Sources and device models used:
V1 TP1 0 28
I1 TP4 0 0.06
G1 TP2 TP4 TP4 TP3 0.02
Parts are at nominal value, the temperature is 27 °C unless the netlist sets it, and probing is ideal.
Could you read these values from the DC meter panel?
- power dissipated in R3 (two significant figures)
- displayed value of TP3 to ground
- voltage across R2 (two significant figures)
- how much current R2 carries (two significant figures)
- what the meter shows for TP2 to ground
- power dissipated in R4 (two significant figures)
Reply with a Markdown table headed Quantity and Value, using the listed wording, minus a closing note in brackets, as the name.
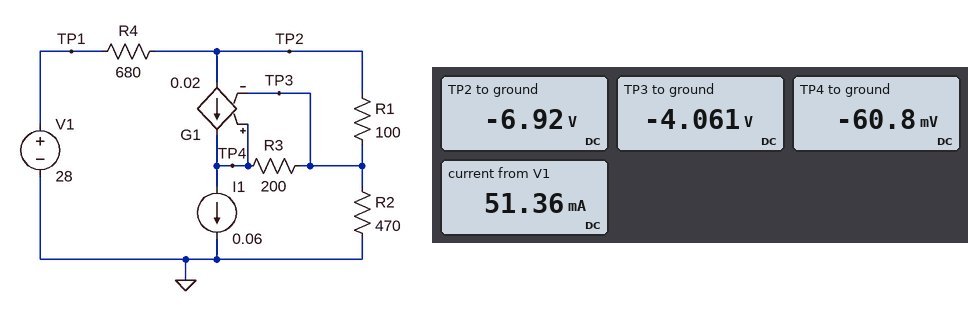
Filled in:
| Quantity | Value |
|---|---|
| power dissipated in R3 | 80 mW |
| displayed value of TP3 to ground | -4.061 V |
| voltage across R2 | 4.1 V |
| how much current R2 carries | 8.6 mA |
| what the meter shows for TP2 to ground | -6.92 V |
| power dissipated in R4 | 1.8 W |
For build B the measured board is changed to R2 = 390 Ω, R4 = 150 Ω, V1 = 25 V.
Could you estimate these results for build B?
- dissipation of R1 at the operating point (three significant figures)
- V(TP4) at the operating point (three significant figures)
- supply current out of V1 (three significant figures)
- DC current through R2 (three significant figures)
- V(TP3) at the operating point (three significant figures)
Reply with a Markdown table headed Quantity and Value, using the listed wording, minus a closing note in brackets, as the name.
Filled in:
| Quantity | Value |
|---|---|
| dissipation of R1 at the operating point | 6.60 mW |
| V(TP4) at the operating point | 15.0 V |
| supply current out of V1 | 88.1 mA |
| DC current through R2 | 28.1 mA |
| V(TP3) at the operating point | 11.0 V |
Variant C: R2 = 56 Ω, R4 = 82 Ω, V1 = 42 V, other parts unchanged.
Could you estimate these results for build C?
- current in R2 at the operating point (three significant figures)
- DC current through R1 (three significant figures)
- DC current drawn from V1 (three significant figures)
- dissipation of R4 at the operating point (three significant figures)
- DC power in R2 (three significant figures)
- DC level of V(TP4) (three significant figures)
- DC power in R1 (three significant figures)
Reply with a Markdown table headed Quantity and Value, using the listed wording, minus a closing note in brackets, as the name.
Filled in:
| Quantity | Value |
|---|---|
| current in R2 at the operating point | 164 mA |
| DC current through R1 | 144 mA |
| DC current drawn from V1 | 224 mA |
| dissipation of R4 at the operating point | 4.12 W |
| DC power in R2 | 1.51 W |
| DC level of V(TP4) | 13.2 V |
| DC power in R1 | 2.08 W |
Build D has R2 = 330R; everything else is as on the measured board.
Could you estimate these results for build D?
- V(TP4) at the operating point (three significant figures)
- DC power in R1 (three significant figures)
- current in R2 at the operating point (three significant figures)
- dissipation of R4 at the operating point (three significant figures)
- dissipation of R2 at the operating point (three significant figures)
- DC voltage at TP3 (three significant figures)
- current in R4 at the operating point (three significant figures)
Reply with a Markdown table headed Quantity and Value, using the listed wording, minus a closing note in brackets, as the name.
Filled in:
| Quantity | Value |
|---|---|
| V(TP4) at the operating point | 789 mV |
| DC power in R1 | 88.4 mW |
| current in R2 at the operating point | 9.73 mA |
| dissipation of R4 at the operating point | 1.72 W |
| dissipation of R2 at the operating point | 31.2 mW |
| DC voltage at TP3 | -3.21 V |
| current in R4 at the operating point | 50.3 mA |
